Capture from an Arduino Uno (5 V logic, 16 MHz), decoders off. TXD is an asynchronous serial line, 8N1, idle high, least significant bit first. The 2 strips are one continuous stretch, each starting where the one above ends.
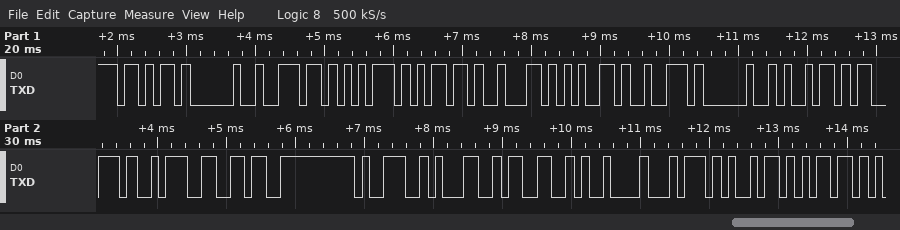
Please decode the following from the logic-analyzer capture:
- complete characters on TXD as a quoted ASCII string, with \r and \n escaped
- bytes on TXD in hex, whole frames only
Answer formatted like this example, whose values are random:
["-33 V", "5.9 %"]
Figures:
["\"k number is:6913\\ttim\"", "6B 20 6E 75 6D 62 65 72 20 69 73 3A 36 39 31 33 09 74 69 6D"]
